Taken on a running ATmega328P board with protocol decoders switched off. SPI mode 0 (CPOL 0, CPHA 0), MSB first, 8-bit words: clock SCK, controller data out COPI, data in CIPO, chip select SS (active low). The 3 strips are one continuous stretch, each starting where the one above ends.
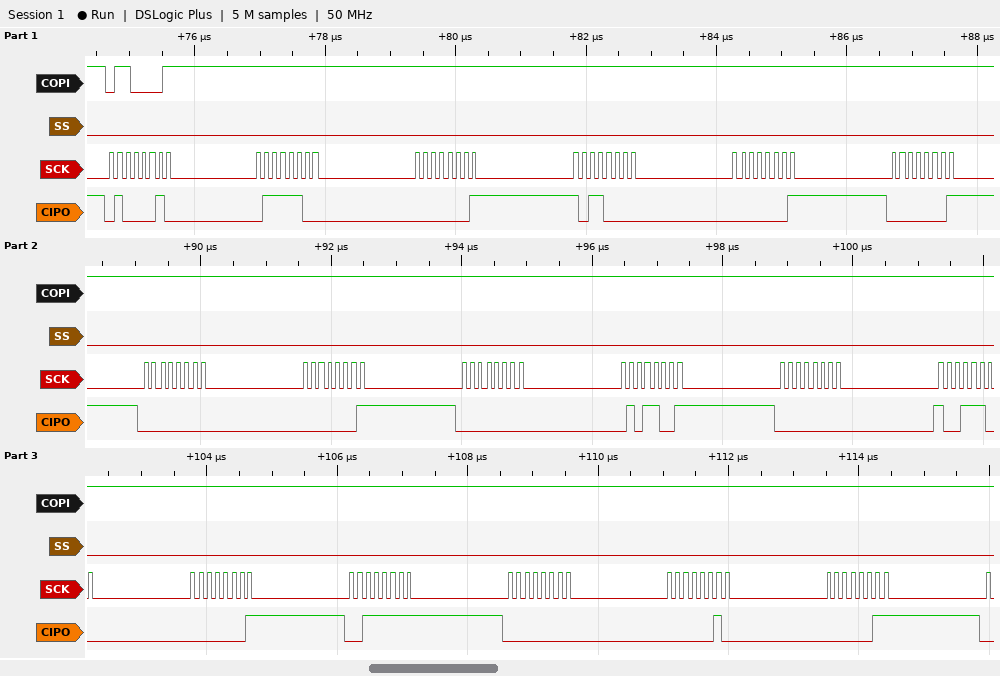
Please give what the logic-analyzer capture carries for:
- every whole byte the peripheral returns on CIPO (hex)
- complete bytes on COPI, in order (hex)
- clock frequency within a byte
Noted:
42 7C 01 B0 01 01 00 01 00 59 00 9C 01 3F 00 02 03
61 FF FF FF FF FF FF FF FF FF FF FF FF FF FF FF FF
8 MHz
